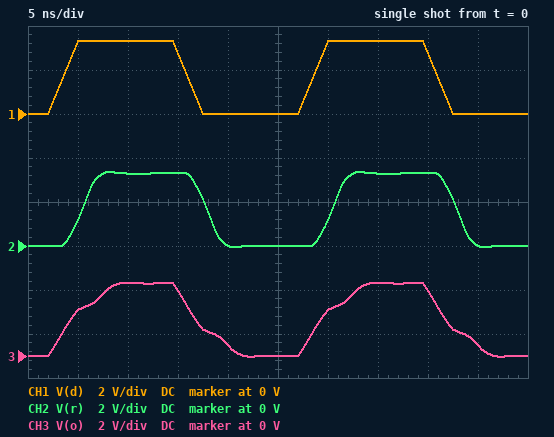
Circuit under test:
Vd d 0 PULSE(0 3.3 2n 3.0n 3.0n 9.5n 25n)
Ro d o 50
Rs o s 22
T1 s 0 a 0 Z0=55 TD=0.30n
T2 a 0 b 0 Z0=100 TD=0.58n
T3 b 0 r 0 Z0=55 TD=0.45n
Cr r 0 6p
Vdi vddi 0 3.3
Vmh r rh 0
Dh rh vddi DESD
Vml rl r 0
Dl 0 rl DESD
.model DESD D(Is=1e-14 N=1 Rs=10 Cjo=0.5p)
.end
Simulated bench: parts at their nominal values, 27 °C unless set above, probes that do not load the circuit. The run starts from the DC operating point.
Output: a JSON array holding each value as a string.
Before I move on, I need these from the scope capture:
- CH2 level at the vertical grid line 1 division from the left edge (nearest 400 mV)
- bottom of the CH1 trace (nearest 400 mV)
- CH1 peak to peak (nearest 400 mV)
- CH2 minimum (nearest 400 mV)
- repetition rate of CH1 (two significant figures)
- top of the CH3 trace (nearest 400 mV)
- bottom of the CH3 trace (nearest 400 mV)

["1.2 V", "0 V", "3.2 V", "0 V", "40 MHz", "3.2 V", "0 V"]
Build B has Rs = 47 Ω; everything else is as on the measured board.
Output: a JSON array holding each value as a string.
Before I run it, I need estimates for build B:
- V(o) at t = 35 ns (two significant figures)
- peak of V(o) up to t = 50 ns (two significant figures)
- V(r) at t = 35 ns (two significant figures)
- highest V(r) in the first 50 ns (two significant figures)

["3.2 V", "3.3 V", "3.1 V", "3.3 V"]
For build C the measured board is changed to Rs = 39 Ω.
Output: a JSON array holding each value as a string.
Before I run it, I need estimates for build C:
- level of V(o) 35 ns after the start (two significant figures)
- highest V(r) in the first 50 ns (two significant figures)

["3.2 V", "3.3 V"]
